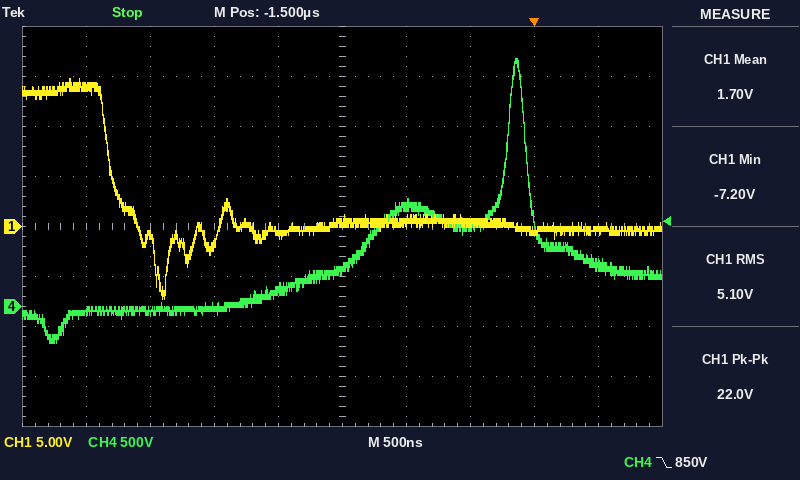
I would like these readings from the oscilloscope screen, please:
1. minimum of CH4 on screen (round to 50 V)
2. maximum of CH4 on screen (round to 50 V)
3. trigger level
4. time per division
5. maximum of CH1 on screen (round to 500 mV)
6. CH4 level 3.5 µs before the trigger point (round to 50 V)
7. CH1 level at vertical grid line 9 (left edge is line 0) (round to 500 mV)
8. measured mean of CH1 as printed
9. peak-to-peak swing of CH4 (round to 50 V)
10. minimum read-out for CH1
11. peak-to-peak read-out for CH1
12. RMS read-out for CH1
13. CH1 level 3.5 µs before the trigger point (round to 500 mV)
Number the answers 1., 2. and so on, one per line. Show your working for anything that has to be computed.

1. -350 V
2. 2.50 kV
3. 850 V
4. 500 ns
5. 15.0 V
6. -50 V
7. -500 mV
8. 1.70 V
9. 2.50 kV − (-350 V) = 2.85 kV
10. -7.20 V
11. 22.0 V
12. 5.10 V
13. 14.0 V
